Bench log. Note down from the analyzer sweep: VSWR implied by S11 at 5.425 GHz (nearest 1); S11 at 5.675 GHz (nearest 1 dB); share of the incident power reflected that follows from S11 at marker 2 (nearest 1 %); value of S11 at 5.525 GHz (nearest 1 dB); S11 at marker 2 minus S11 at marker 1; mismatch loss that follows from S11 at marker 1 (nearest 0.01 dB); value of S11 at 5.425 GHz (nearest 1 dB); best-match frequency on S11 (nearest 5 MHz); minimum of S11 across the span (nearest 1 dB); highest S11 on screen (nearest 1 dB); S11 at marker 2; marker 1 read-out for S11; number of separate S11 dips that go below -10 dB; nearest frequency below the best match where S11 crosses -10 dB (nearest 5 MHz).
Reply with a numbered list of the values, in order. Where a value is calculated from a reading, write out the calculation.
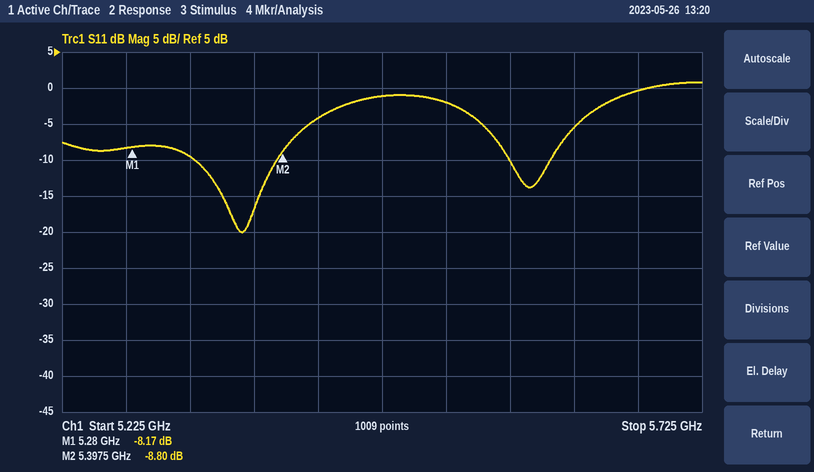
1. |Γ| = 10^(-4/20) = 0.6310; VSWR = (1 + 0.6310)/(1 − 0.6310) ≈ 4
2. 0 dB
3. 10^(-8.8/10) ≈ 13 %
4. -2 dB
5. -8.8 − (-8.17) = -0.63 dB
6. −10 log10(1 − 10^(-8.17/10)) ≈ 0.72 dB
7. -4 dB
8. 5.365 GHz
9. -20 dB
10. 1 dB
11. -8.80 dB
12. -8.17 dB
13. 2
14. 5.330 GHz
